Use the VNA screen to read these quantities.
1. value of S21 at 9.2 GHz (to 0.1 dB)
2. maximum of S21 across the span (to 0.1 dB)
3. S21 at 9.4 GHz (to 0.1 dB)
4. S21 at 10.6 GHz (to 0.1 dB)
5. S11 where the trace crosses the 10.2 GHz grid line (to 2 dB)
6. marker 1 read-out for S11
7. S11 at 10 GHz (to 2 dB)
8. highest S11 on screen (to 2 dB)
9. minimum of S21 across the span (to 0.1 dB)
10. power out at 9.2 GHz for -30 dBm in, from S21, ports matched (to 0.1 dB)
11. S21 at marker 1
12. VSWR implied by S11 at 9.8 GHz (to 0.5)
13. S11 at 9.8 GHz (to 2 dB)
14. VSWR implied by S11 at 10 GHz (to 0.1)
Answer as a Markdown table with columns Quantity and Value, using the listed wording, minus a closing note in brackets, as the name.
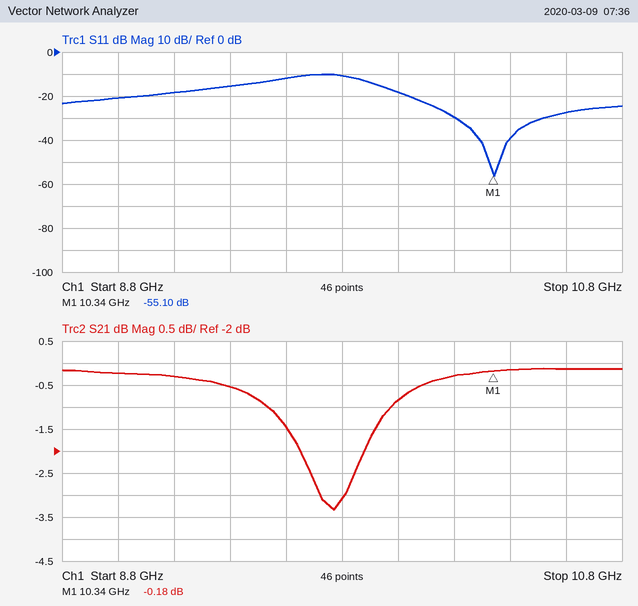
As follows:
| Quantity | Value |
|---|---|
| value of S21 at 9.2 GHz | -0.3 dB |
| maximum of S21 across the span | -0.1 dB |
| S21 at 9.4 GHz | -0.5 dB |
| S21 at 10.6 GHz | -0.1 dB |
| S11 where the trace crosses the 10.2 GHz grid line | -30 dB |
| marker 1 read-out for S11 | -55.10 dB |
| S11 at 10 GHz | -18 dB |
| highest S11 on screen | -10 dB |
| minimum of S21 across the span | -3.3 dB |
| power out at 9.2 GHz for -30 dBm in, from S21, ports matched | -30.3 dBm |
| S21 at marker 1 | -0.18 dB |
| VSWR implied by S11 at 9.8 GHz | 2.0 |
| S11 at 9.8 GHz | -10 dB |
| VSWR implied by S11 at 10 GHz | 1.3 |
